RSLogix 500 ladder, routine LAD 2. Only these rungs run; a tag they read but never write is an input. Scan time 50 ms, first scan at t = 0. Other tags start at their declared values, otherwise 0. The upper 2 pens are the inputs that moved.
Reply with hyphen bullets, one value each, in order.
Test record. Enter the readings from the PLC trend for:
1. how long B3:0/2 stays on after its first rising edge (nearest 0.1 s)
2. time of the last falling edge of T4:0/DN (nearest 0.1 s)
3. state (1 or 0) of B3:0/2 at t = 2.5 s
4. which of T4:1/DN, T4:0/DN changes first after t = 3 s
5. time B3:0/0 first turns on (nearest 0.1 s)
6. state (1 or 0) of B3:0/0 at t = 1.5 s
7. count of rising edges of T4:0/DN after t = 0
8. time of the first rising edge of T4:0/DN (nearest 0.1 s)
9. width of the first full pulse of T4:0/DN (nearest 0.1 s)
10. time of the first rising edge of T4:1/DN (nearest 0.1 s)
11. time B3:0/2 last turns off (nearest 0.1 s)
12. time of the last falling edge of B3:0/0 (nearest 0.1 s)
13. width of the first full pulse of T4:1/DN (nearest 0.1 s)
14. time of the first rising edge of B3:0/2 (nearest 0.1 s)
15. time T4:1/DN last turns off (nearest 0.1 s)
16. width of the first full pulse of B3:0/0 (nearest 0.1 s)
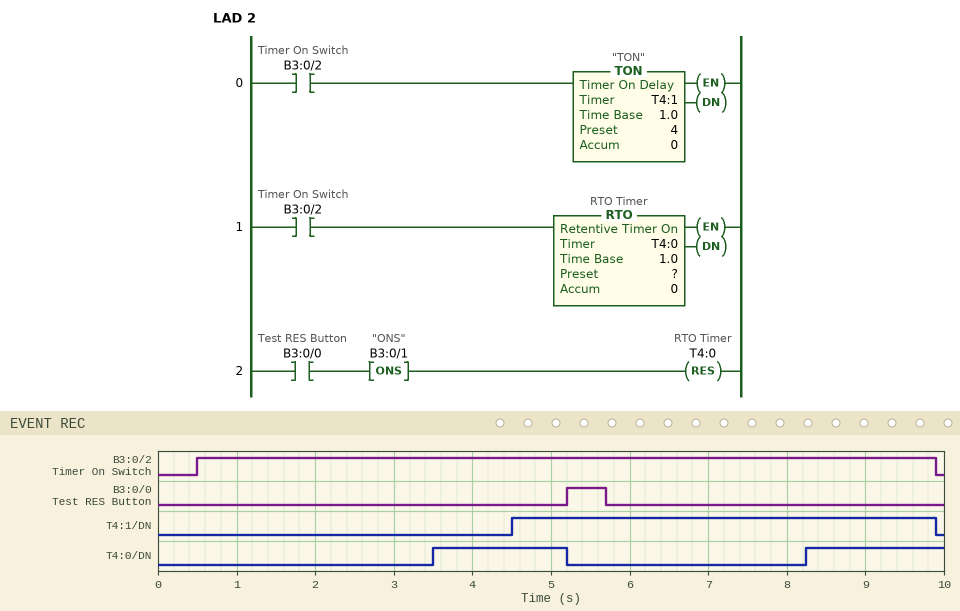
- 9.4 s
- 5.2 s
- 1
- T4:0/DN
- 5.2 s
- 0
- 2
- 3.5 s
- 1.7 s
- 4.5 s
- 9.9 s
- 5.7 s
- 5.4 s
- 0.5 s
- 9.9 s
- 0.5 s
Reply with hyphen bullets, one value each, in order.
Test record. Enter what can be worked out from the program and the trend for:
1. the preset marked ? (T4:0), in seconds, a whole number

- 3 s
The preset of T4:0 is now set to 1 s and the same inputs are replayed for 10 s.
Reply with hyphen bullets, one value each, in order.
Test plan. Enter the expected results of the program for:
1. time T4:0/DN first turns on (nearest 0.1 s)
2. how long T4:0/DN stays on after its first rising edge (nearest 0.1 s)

- 1.5 s
- 3.7 s
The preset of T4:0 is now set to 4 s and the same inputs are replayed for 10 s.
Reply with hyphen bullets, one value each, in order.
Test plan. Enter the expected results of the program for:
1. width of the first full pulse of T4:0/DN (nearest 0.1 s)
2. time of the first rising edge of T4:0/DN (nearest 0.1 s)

- 0.7 s
- 4.5 s
